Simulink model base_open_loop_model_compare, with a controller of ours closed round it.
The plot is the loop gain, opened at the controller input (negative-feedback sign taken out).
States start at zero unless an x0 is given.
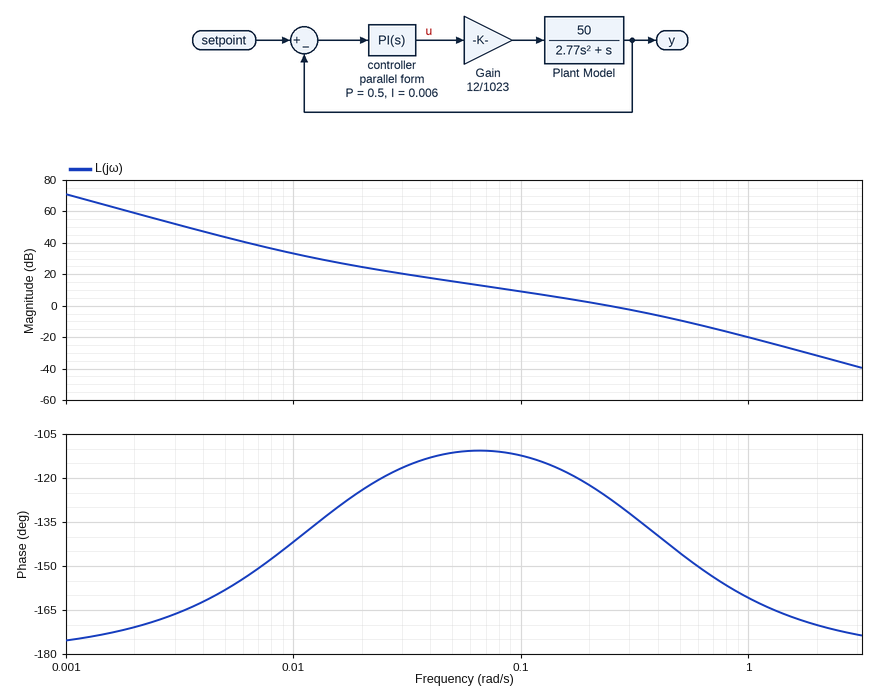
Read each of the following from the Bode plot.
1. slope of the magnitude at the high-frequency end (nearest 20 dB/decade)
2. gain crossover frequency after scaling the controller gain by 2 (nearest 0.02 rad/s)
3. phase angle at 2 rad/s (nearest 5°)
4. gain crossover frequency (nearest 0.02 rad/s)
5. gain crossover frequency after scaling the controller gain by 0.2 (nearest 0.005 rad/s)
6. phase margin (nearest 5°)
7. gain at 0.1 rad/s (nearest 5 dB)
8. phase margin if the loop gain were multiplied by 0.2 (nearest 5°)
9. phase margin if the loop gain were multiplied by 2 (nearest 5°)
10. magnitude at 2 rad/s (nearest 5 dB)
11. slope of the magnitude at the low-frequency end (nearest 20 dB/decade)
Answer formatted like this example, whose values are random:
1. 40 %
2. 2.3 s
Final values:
1. -40 dB/decade
2. 0.40 rad/s
3. -170°
4. 0.24 rad/s
5. 0.060 rad/s
6. 55°
7. 10 dB
8. 70°
9. 40°
10. -30 dB
11. -40 dB/decade
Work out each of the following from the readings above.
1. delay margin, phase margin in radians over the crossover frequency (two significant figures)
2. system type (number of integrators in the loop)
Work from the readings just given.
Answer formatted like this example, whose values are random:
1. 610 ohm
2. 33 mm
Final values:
1. 4.0 s
2. 2
